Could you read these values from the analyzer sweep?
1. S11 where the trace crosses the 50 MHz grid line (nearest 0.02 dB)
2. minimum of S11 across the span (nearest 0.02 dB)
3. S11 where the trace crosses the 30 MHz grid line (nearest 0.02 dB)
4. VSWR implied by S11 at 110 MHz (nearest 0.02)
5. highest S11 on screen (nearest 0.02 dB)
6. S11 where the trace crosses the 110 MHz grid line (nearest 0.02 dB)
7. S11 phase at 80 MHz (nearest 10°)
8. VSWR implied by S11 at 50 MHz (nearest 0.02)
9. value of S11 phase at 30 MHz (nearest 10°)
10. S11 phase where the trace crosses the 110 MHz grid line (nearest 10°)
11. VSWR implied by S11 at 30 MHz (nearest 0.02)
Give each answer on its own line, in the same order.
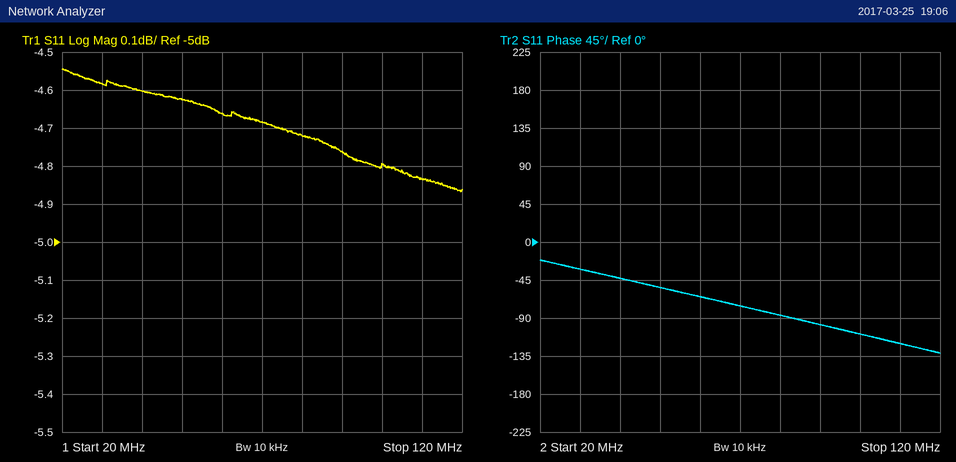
-4.62 dB
-4.86 dB
-4.58 dB
3.68
-4.54 dB
-4.84 dB
-90°
3.84
-30°
-120°
3.88
